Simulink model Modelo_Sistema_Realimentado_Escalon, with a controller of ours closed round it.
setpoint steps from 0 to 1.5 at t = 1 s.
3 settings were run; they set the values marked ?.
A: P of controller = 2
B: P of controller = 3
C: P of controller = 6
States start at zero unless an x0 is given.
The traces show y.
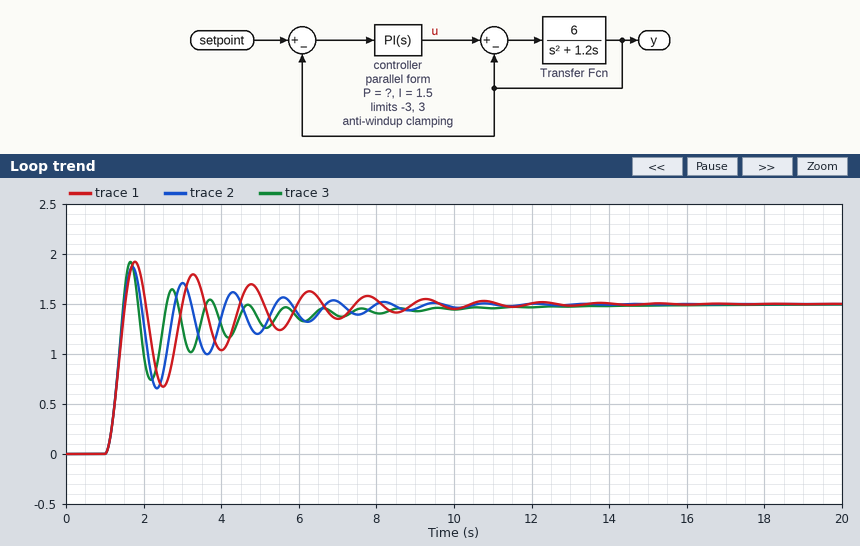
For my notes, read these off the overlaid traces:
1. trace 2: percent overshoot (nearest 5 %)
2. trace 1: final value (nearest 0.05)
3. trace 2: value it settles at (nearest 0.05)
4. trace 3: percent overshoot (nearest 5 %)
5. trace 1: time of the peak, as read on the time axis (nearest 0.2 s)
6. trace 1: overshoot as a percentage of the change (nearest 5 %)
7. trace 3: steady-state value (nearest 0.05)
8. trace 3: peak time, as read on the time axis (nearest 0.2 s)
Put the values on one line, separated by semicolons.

25 %; 1.50; 1.50; 30 %; 1.8 s; 30 %; 1.50; 1.6 s
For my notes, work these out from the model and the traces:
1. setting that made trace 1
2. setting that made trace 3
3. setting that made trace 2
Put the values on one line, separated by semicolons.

A; C; B
